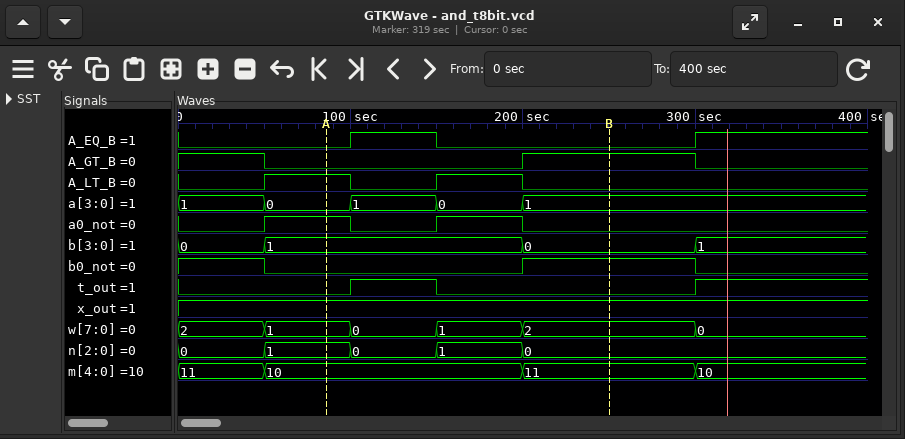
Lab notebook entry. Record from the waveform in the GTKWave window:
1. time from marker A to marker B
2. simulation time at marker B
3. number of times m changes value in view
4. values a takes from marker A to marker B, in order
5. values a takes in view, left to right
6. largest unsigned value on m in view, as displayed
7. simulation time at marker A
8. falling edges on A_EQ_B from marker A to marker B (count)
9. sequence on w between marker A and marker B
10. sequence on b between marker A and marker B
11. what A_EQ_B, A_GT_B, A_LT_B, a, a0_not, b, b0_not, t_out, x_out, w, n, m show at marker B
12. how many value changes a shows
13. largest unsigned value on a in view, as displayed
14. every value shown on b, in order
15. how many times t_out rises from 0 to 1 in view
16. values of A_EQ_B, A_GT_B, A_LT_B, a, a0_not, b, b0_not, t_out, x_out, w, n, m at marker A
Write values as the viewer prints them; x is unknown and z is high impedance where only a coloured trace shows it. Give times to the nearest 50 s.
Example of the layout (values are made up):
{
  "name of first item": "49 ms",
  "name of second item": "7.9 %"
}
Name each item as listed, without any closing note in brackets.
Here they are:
{
  "time from marker A to marker B": "150 s",
  "simulation time at marker B": "250 s",
  "number of times m changes value in view": "3",
  "values a takes from marker A to marker B, in order": "0, 1, 0, 1",
  "values a takes in view, left to right": "1, 0, 1, 0, 1",
  "largest unsigned value on m in view, as displayed": "11",
  "simulation time at marker A": "100 s",
  "falling edges on A_EQ_B from marker A to marker B": "1",
  "sequence on w between marker A and marker B": "1, 0, 1, 2",
  "sequence on b between marker A and marker B": "1, 0",
  "what A_EQ_B, A_GT_B, A_LT_B, a, a0_not, b, b0_not, t_out, x_out, w, n, m show at marker B": "A_EQ_B=0, A_GT_B=1, A_LT_B=0, a=1, a0_not=0, b=0, b0_not=1, t_out=0, x_out=1, w=2, n=0, m=11",
  "how many value changes a shows": "4",
  "largest unsigned value on a in view, as displayed": "1",
  "every value shown on b, in order": "0, 1, 0, 1",
  "how many times t_out rises from 0 to 1 in view": "2",
  "values of A_EQ_B, A_GT_B, A_LT_B, a, a0_not, b, b0_not, t_out, x_out, w, n, m at marker A": "A_EQ_B=0, A_GT_B=0, A_LT_B=1, a=0, a0_not=1, b=1, b0_not=0, t_out=0, x_out=1, w=1, n=1, m=10"
}
